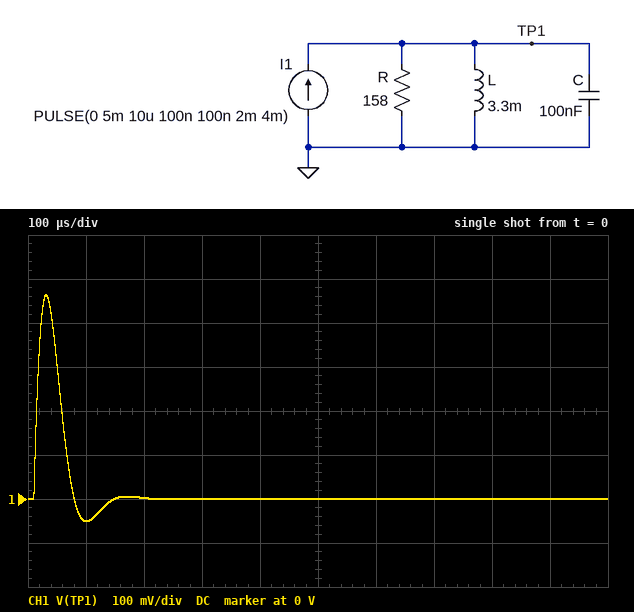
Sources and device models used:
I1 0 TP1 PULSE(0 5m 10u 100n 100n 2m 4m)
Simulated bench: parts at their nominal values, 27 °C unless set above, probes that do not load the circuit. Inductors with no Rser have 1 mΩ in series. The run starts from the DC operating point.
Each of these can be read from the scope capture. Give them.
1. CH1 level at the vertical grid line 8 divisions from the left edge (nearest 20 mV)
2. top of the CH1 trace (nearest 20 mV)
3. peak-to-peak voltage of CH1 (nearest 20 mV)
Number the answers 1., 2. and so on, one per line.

1. 0 V
2. 460 mV
3. 520 mV
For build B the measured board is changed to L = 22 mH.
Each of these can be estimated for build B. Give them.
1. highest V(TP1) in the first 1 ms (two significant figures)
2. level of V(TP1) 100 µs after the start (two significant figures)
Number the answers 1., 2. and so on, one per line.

1. 650 mV
2. 500 mV
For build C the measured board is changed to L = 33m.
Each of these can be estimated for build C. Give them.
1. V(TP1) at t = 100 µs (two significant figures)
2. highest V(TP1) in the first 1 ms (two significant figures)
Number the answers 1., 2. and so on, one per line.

1. 590 mV
2. 680 mV
